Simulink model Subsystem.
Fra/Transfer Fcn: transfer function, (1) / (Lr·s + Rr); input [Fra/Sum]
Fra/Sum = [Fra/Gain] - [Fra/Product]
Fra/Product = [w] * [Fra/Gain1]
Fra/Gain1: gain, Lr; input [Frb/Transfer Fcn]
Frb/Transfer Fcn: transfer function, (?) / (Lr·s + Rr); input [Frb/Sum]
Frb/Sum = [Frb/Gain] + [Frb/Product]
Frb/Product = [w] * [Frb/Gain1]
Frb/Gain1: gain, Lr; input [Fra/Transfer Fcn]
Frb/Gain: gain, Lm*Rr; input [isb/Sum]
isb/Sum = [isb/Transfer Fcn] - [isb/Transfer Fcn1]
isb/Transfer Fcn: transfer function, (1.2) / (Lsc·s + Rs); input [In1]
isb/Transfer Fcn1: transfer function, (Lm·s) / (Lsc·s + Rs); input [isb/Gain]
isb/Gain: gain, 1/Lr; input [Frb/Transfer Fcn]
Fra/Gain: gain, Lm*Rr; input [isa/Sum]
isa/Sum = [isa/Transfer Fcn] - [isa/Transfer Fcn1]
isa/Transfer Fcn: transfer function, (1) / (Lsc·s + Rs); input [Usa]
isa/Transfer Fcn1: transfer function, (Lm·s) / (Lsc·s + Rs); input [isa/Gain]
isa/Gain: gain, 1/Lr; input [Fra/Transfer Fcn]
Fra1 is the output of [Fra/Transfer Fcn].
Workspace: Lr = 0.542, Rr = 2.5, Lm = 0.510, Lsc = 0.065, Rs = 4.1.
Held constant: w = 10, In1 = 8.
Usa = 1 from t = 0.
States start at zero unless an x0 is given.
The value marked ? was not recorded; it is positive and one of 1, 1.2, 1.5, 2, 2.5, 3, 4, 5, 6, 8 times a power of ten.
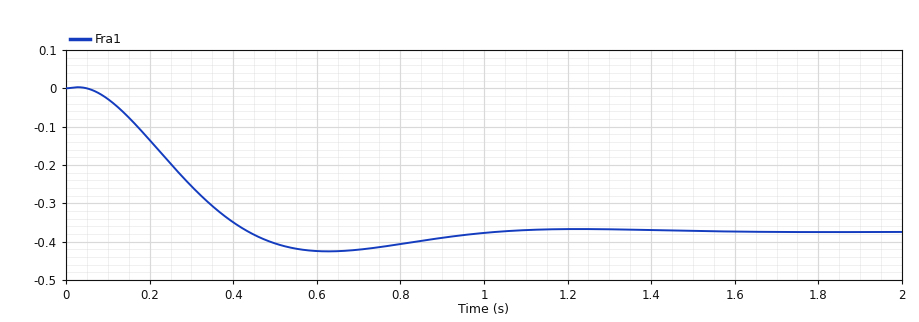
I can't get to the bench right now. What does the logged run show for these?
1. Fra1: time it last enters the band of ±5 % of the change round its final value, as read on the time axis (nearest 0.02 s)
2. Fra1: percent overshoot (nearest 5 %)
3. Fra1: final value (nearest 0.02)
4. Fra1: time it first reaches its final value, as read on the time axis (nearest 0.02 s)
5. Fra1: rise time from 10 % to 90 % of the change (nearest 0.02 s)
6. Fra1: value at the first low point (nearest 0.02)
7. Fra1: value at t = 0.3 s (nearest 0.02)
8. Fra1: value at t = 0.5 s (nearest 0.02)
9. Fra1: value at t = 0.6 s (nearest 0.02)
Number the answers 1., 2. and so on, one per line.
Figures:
1. 0.88 s
2. 15 %
3. -0.38
4. 0.44 s
5. 0.28 s
6. -0.42
7. -0.26
8. -0.40
9. -0.42
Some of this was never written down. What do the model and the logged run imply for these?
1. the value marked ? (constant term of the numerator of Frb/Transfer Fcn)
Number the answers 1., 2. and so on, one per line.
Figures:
1. 0.6
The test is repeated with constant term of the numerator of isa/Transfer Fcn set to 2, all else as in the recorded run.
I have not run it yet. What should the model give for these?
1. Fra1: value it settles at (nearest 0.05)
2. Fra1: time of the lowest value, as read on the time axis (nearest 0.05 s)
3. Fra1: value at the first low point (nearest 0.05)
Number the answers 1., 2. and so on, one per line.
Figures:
1. -0.35
2. 0.65 s
3. -0.40
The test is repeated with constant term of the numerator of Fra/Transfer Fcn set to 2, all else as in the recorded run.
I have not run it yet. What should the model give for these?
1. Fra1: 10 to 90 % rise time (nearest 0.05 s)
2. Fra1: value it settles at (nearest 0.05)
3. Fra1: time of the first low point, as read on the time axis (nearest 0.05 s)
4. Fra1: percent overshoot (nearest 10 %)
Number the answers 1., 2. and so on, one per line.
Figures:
1. 0.20 s
2. -0.45
3. 0.50 s
4. 20 %
